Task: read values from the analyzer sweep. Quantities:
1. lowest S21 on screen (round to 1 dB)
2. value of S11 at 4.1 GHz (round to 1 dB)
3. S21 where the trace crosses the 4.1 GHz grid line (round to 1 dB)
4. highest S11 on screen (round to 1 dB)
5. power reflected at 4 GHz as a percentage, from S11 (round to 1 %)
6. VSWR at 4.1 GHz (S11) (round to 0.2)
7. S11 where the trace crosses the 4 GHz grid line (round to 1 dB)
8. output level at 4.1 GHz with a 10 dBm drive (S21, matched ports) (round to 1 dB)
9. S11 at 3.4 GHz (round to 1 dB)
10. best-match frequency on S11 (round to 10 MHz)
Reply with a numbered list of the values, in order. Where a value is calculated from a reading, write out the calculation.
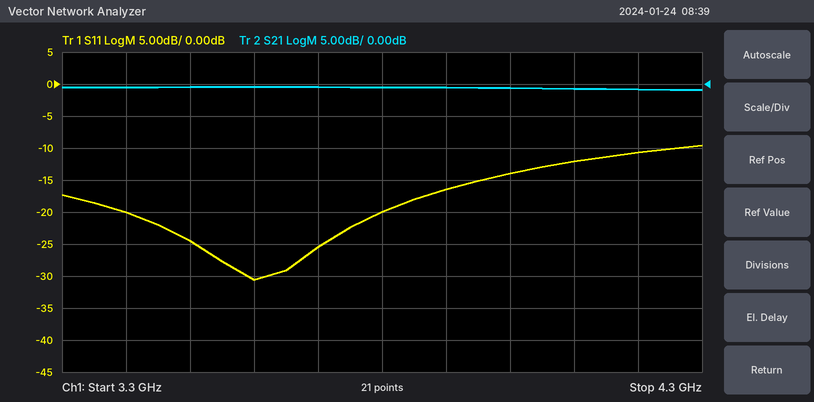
1. -1 dB
2. -12 dB
3. -1 dB
4. -10 dB
5. 10^(-14/10) ≈ 4 %
6. |Γ| = 10^(-12/20) = 0.2512; VSWR = (1 + 0.2512)/(1 − 0.2512) ≈ 1.67, so 1.6 to the nearest 0.2
7. -14 dB
8. 10 dBm + (-1 dB) = 9 dBm
9. -20 dB
10. 3.60 GHz
